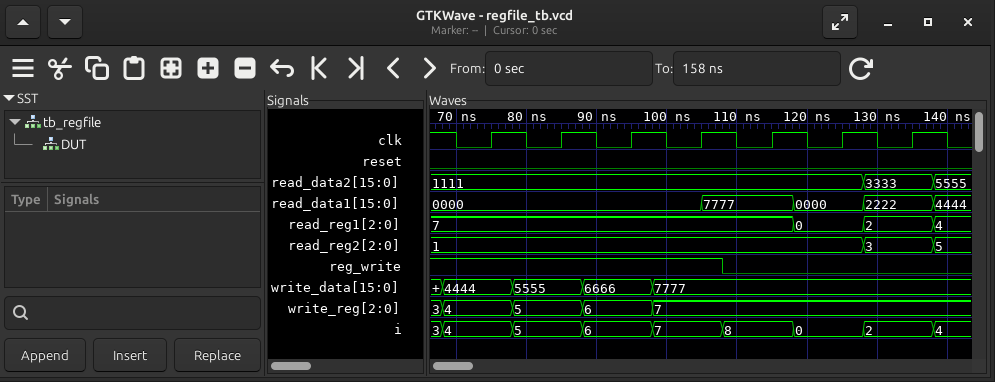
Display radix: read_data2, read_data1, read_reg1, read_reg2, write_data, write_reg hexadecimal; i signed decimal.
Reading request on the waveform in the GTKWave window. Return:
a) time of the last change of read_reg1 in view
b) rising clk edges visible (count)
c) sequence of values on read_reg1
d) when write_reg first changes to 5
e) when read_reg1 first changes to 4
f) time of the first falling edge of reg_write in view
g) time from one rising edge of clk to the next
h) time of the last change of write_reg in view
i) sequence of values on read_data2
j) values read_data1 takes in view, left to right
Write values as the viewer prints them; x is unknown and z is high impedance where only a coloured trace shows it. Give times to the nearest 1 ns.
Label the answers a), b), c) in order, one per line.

a) 138 ns
b) 7
c) 7, 0, 2, 4
d) 78 ns
e) 138 ns
f) 108 ns
g) 10 ns
h) 98 ns
i) 1111, 3333, 5555
j) 0000, 7777, 0000, 2222, 4444
